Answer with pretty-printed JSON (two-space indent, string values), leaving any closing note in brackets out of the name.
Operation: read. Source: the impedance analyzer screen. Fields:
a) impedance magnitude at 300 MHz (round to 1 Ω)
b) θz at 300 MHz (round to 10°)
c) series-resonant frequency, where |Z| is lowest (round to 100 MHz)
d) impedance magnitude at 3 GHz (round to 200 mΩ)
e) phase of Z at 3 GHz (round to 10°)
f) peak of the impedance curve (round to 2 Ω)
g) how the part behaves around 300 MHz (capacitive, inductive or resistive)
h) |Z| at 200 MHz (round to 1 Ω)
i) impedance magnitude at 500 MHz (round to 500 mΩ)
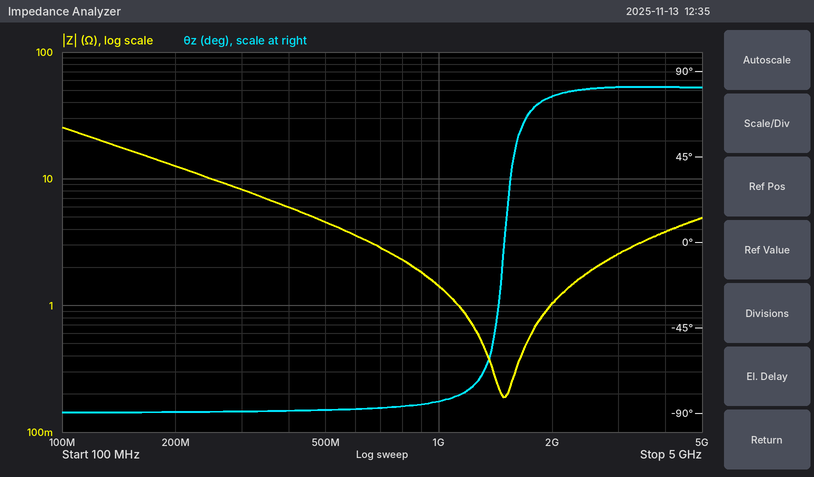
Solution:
{
  "impedance magnitude at 300 MHz": "8 Ω",
  "θz at 300 MHz": "-90°",
  "series-resonant frequency, where |Z| is lowest": "1.5 GHz",
  "impedance magnitude at 3 GHz": "2.6 Ω",
  "phase of Z at 3 GHz": "80°",
  "peak of the impedance curve": "26 Ω",
  "how the part behaves around 300 MHz": "capacitive",
  "|Z| at 200 MHz": "13 Ω",
  "impedance magnitude at 500 MHz": "4.5 Ω"
}
